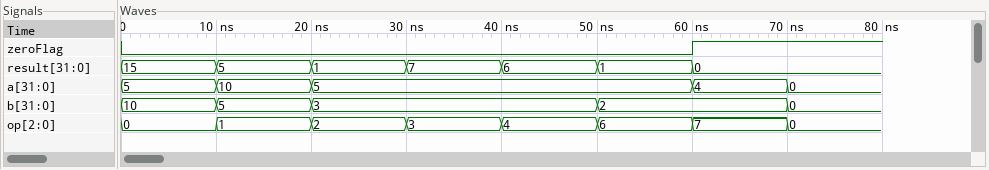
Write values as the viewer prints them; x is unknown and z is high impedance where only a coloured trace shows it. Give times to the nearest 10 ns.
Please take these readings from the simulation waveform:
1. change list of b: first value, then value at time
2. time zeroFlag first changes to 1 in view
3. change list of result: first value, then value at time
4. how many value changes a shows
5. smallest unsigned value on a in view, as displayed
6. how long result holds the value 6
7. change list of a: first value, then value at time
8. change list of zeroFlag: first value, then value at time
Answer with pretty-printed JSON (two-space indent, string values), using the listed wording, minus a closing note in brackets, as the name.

{
  "change list of b: first value, then value at time": "10, 5 at 10 ns, 3 at 20 ns, 2 at 50 ns, 0 at 70 ns",
  "time zeroFlag first changes to 1 in view": "60 ns",
  "change list of result: first value, then value at time": "15, 5 at 10 ns, 1 at 20 ns, 7 at 30 ns, 6 at 40 ns, 1 at 50 ns, 0 at 60 ns",
  "how many value changes a shows": "4",
  "smallest unsigned value on a in view, as displayed": "0",
  "how long result holds the value 6": "10 ns",
  "change list of a: first value, then value at time": "5, 10 at 10 ns, 5 at 20 ns, 4 at 60 ns, 0 at 70 ns",
  "change list of zeroFlag: first value, then value at time": "0, 1 at 60 ns"
}
